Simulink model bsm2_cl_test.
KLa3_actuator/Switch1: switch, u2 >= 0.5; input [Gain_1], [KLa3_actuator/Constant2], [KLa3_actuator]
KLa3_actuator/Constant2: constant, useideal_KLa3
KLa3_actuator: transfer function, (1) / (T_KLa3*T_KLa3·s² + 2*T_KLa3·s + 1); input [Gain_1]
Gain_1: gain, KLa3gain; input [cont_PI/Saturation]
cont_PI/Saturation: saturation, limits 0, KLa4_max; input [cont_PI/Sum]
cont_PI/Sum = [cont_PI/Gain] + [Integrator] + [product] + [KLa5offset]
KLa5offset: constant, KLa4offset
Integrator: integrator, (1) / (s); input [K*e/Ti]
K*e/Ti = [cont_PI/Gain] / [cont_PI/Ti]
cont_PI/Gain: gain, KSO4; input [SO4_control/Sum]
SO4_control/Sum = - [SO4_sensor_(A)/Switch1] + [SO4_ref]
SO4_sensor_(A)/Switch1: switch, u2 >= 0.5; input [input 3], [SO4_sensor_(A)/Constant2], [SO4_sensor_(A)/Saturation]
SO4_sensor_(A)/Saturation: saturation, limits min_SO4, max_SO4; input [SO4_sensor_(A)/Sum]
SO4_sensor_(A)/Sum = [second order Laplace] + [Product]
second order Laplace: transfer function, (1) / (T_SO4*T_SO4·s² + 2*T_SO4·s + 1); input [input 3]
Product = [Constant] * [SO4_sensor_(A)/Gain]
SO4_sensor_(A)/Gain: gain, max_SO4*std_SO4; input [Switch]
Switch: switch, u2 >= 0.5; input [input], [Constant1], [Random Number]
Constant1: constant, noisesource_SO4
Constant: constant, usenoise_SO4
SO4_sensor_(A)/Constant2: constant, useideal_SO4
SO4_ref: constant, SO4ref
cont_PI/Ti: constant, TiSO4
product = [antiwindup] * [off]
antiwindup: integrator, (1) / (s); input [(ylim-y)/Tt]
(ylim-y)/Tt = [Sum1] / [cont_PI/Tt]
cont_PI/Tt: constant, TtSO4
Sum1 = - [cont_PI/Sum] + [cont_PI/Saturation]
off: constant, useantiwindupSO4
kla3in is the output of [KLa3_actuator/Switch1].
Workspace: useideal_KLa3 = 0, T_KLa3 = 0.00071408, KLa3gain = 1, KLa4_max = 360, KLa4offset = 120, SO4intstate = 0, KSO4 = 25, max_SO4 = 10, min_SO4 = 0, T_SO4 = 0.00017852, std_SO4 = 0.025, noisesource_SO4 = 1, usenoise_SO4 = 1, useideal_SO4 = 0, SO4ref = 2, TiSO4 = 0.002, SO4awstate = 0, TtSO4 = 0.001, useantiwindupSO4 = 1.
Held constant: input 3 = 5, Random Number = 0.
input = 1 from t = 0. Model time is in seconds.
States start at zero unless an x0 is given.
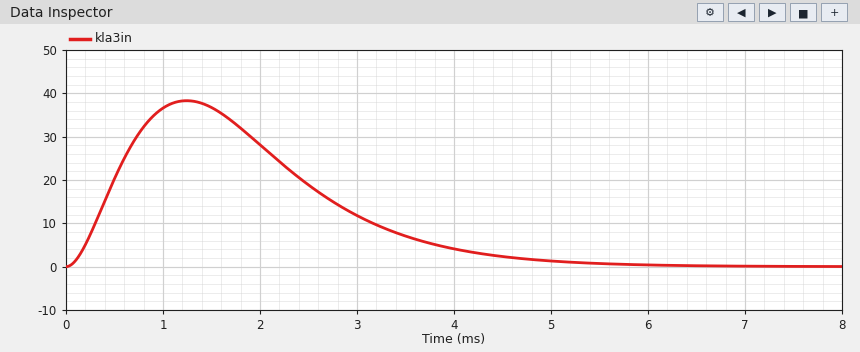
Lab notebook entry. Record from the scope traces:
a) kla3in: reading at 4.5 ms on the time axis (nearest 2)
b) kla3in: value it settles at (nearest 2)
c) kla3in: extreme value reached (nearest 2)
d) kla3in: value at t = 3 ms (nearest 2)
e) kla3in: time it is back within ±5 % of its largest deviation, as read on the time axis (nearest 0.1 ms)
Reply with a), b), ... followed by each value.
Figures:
a) 2
b) 0
c) 38
d) 12
e) 4.7 ms
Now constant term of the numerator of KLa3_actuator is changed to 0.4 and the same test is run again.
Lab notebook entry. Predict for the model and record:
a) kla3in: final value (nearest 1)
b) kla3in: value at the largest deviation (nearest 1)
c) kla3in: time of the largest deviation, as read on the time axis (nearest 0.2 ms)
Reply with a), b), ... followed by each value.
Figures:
a) 0
b) 15
c) 1.2 ms
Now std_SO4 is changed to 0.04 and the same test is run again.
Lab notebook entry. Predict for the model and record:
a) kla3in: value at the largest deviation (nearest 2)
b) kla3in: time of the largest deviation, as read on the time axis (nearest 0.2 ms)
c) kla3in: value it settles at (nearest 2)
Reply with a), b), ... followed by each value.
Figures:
a) 36
b) 1.2 ms
c) 0
